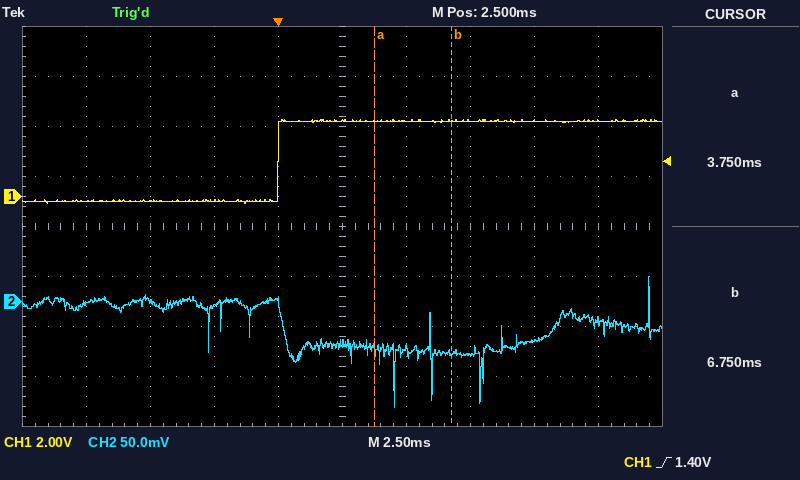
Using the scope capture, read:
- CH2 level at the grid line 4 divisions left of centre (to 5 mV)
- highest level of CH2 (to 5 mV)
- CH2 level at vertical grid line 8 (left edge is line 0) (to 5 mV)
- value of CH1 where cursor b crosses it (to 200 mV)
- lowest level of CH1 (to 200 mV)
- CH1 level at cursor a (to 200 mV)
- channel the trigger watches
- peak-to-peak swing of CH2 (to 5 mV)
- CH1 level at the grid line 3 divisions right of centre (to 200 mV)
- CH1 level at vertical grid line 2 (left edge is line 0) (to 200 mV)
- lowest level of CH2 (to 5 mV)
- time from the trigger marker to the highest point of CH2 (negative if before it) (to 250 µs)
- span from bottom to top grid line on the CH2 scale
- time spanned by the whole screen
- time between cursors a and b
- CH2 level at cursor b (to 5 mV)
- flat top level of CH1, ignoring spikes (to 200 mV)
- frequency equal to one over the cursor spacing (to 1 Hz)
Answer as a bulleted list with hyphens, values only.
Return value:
- 0 mV
- 25 mV
- -40 mV
- 3.0 V
- -200 mV
- 3.0 V
- CH1
- 130 mV
- 3.0 V
- -200 mV
- -105 mV
- +14.50 ms
- 400 mV
- 25 ms
- 3.00 ms
- -50 mV
- 3.0 V
- 333 Hz
